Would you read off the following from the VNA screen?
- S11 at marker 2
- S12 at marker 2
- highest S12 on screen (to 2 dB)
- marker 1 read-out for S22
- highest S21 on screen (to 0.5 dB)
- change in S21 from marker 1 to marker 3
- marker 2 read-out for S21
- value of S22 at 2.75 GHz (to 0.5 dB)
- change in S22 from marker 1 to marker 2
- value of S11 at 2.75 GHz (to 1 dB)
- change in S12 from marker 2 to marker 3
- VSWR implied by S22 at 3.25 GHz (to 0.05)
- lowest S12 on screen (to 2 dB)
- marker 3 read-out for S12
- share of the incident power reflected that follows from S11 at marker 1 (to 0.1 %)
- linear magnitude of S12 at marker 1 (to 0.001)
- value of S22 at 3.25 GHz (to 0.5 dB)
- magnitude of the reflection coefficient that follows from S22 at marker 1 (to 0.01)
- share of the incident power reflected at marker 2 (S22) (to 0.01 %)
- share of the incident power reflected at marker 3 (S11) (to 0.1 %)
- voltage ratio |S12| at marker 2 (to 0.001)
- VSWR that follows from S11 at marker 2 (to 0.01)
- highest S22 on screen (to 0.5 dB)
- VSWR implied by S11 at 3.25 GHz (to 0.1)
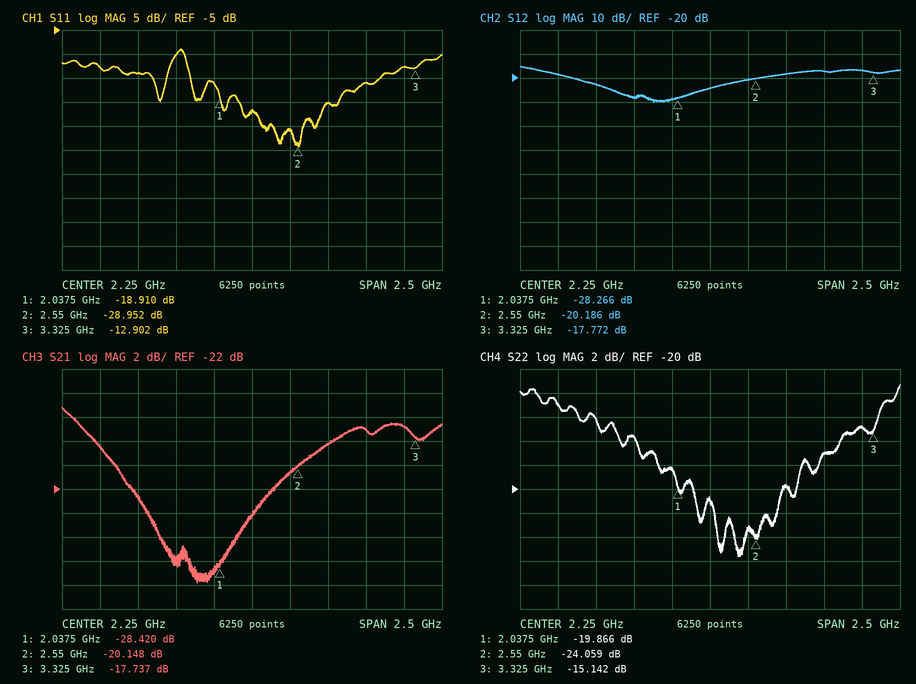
-28.952 dB
-20.186 dB
-16 dB
-19.866 dB
-15.0 dB
10.683 dB
-20.148 dB
-20.0 dB
-4.193 dB
-20 dB
2.414 dB
1.45
-30 dB
-17.772 dB
1.3 %
0.039
-15.0 dB
0.10
0.39 %
5.1 %
0.098
1.07
-11.5 dB
1.6
